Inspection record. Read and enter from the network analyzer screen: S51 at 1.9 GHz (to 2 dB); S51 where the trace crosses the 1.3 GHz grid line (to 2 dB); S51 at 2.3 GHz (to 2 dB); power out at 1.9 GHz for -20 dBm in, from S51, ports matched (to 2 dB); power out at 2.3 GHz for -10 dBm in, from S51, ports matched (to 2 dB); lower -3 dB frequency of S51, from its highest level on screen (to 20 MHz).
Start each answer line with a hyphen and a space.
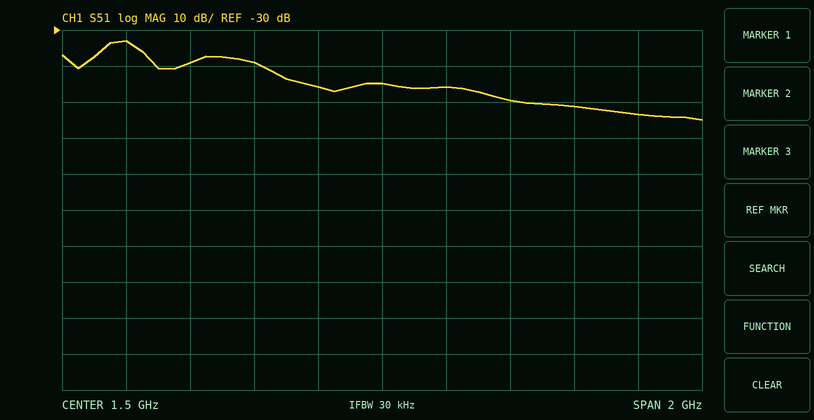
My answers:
- -50 dB
- -46 dB
- -54 dB
- -70 dBm
- -64 dBm
- 620 MHz
